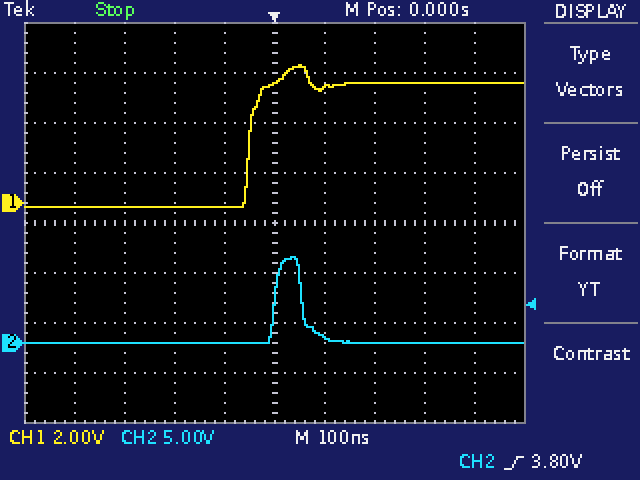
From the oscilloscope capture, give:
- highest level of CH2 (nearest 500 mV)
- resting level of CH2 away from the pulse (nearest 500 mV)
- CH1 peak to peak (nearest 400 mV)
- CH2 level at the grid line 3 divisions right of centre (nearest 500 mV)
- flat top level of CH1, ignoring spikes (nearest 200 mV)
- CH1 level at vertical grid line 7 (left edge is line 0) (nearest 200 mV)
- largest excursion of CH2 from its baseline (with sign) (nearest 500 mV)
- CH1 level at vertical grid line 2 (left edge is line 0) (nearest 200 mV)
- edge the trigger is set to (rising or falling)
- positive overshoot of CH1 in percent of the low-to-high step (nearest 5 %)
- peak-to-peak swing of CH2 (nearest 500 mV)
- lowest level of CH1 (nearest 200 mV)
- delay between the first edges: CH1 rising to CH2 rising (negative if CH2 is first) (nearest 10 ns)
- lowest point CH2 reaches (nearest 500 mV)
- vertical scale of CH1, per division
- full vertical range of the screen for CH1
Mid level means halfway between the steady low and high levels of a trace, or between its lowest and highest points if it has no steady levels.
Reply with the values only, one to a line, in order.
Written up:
8.5 V
0.0 V
5.6 V
0.0 V
4.8 V
4.8 V
+8.5 V
-200 mV
rising
15 %
8.5 V
-200 mV
+50 ns
0.0 V
2 V
16 V
